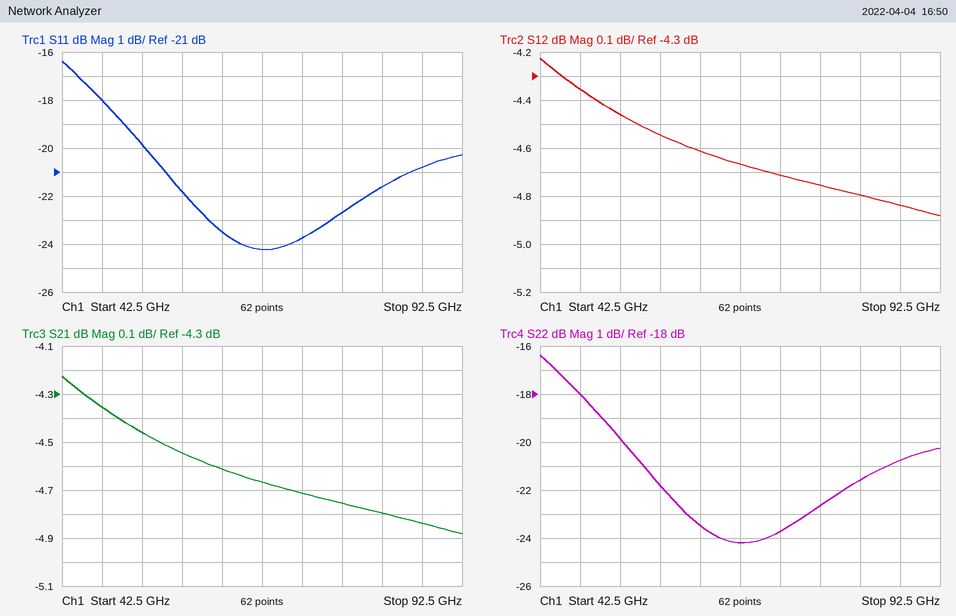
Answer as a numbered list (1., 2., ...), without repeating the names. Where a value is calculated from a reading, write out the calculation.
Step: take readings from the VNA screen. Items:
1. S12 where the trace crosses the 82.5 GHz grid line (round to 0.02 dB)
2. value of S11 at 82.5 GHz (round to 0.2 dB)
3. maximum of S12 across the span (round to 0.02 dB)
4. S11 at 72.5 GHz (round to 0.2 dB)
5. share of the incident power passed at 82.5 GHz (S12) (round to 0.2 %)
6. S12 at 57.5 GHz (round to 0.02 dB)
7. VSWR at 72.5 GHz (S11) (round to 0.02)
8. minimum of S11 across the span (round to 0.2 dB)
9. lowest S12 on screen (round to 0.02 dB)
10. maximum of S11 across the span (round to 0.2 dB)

1. -4.80 dB
2. -21.6 dB
3. -4.22 dB
4. -23.8 dB
5. 10^(-4.8/10) ≈ 33.1 %, so 33.2 % to the nearest 0.2 %
6. -4.54 dB
7. |Γ| = 10^(-23.8/20) = 0.0646; VSWR = (1 + 0.0646)/(1 − 0.0646) ≈ 1.14
8. -24.2 dB
9. -4.88 dB
10. -16.4 dB
